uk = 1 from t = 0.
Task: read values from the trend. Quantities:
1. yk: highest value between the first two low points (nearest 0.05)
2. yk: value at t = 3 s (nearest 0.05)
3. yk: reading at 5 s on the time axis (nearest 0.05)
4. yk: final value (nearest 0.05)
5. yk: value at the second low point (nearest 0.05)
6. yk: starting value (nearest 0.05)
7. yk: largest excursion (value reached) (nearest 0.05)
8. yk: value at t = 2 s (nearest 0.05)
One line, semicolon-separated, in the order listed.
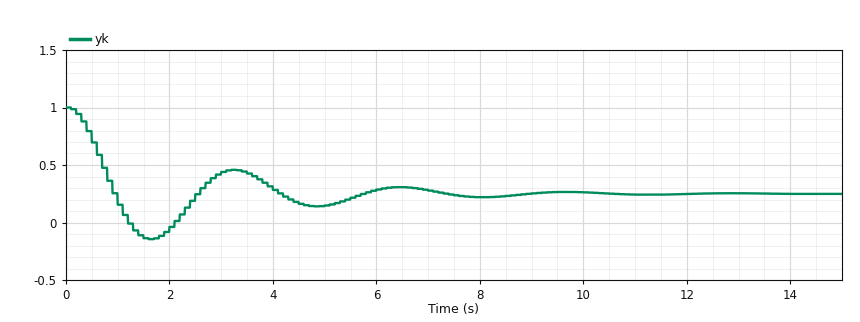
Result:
0.45; 0.45; 0.15; 0.25; 0.15; 1.00; -0.15; -0.05
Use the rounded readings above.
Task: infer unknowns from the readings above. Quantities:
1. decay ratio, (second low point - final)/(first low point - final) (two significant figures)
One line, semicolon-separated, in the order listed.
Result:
0.25
